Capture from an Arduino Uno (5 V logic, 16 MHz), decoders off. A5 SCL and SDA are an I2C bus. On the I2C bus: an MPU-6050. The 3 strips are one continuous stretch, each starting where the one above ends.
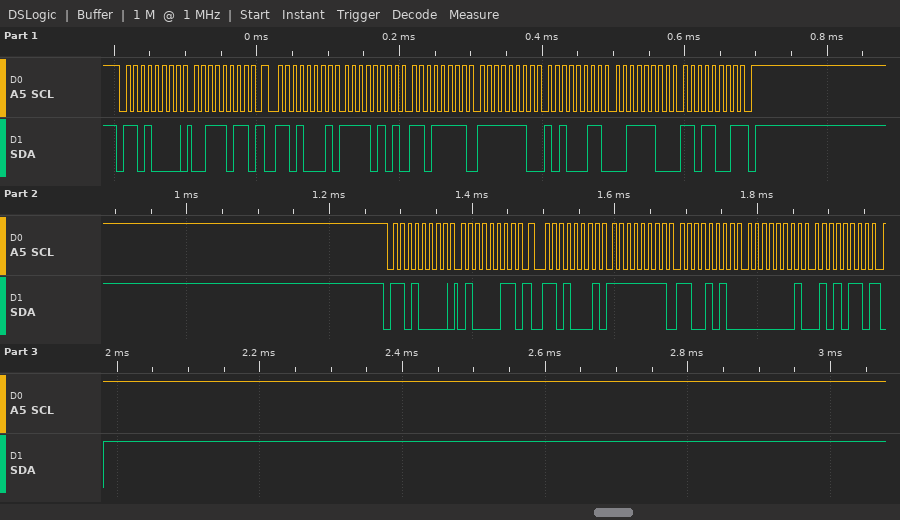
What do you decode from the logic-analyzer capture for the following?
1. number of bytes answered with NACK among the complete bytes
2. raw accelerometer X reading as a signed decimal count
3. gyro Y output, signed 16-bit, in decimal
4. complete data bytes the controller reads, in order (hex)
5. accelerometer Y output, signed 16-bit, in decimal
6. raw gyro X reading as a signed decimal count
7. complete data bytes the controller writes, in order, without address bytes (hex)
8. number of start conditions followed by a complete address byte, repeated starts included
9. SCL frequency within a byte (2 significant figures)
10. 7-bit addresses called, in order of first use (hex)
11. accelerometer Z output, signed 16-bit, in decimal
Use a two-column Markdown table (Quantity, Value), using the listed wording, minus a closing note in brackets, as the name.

| Quantity | Value |
|---|---|
| number of bytes answered with NACK among the complete bytes | 2 |
| raw accelerometer X reading as a signed decimal count | -2593 |
| gyro Y output, signed 16-bit, in decimal | 342 |
| complete data bytes the controller reads, in order | F5 DF FE A3 3C D9 FF CA 01 56 |
| accelerometer Y output, signed 16-bit, in decimal | -349 |
| raw gyro X reading as a signed decimal count | -54 |
| complete data bytes the controller writes, in order, without address bytes | 3B 43 |
| number of start conditions followed by a complete address byte, repeated starts included | 4 |
| SCL frequency within a byte | 100 kHz |
| 7-bit addresses called, in order of first use | 0x68 |
| accelerometer Z output, signed 16-bit, in decimal | 15577 |
